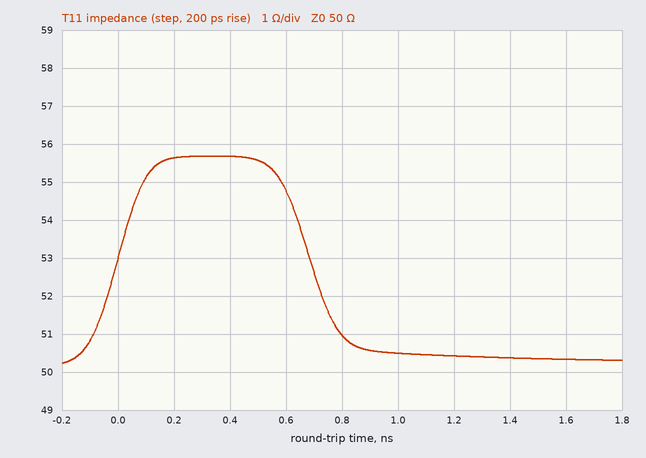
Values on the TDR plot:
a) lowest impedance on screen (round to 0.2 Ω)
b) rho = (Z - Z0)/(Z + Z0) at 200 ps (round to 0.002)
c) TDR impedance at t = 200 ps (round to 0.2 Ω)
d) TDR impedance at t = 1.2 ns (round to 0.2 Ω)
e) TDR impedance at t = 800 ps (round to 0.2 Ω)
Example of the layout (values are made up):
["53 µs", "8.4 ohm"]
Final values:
["50.2 Ω", "+0.054", "55.6 Ω", "50.4 Ω", "51.0 Ω"]
